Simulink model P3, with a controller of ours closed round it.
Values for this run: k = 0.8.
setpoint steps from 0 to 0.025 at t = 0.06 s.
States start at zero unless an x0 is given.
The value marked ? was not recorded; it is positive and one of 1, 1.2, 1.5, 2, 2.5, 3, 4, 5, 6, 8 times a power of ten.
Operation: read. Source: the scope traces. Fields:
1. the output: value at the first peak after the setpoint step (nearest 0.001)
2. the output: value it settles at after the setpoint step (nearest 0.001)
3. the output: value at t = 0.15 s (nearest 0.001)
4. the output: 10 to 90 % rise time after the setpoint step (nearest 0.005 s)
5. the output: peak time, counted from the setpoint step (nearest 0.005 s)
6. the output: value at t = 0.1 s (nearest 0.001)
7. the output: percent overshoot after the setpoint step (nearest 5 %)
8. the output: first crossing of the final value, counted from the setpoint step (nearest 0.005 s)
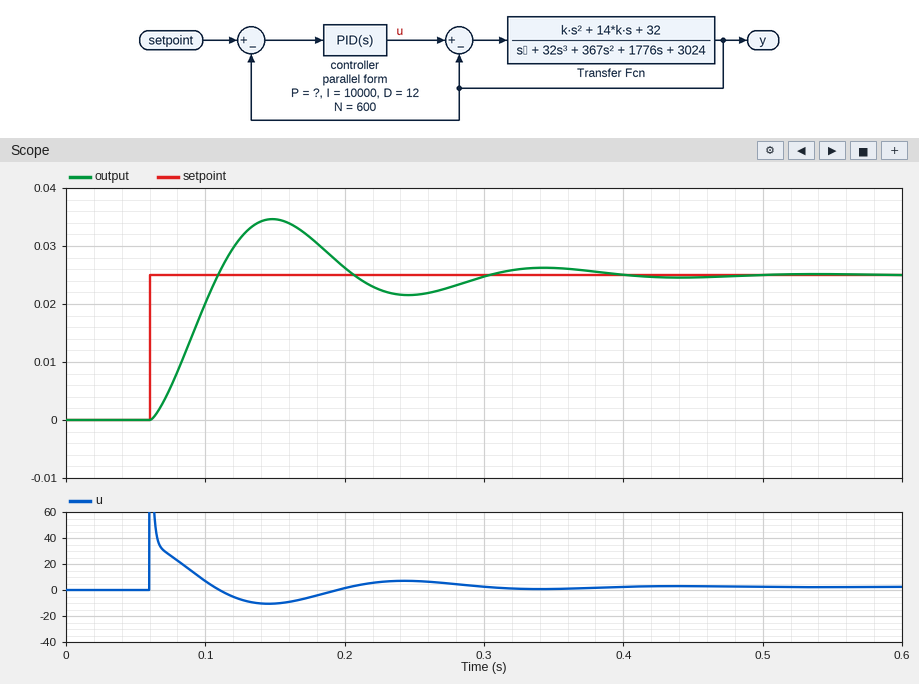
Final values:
0.035
0.025
0.035
0.035 s
0.090 s
0.020
40 %
0.050 s
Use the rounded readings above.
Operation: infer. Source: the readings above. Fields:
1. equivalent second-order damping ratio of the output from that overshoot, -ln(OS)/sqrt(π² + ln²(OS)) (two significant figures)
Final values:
0.28
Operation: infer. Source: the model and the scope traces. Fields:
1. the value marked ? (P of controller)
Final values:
1500
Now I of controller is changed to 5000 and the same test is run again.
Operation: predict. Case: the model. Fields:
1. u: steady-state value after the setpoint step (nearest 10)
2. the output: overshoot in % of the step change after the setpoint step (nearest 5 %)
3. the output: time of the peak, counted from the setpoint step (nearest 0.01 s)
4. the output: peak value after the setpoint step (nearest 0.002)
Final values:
0
30 %
0.09 s
0.032
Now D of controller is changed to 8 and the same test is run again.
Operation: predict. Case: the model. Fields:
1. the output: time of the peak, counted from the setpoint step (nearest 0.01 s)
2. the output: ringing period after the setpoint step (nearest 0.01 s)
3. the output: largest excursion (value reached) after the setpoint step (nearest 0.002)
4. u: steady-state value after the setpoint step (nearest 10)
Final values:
0.09 s
0.19 s
0.036
0
